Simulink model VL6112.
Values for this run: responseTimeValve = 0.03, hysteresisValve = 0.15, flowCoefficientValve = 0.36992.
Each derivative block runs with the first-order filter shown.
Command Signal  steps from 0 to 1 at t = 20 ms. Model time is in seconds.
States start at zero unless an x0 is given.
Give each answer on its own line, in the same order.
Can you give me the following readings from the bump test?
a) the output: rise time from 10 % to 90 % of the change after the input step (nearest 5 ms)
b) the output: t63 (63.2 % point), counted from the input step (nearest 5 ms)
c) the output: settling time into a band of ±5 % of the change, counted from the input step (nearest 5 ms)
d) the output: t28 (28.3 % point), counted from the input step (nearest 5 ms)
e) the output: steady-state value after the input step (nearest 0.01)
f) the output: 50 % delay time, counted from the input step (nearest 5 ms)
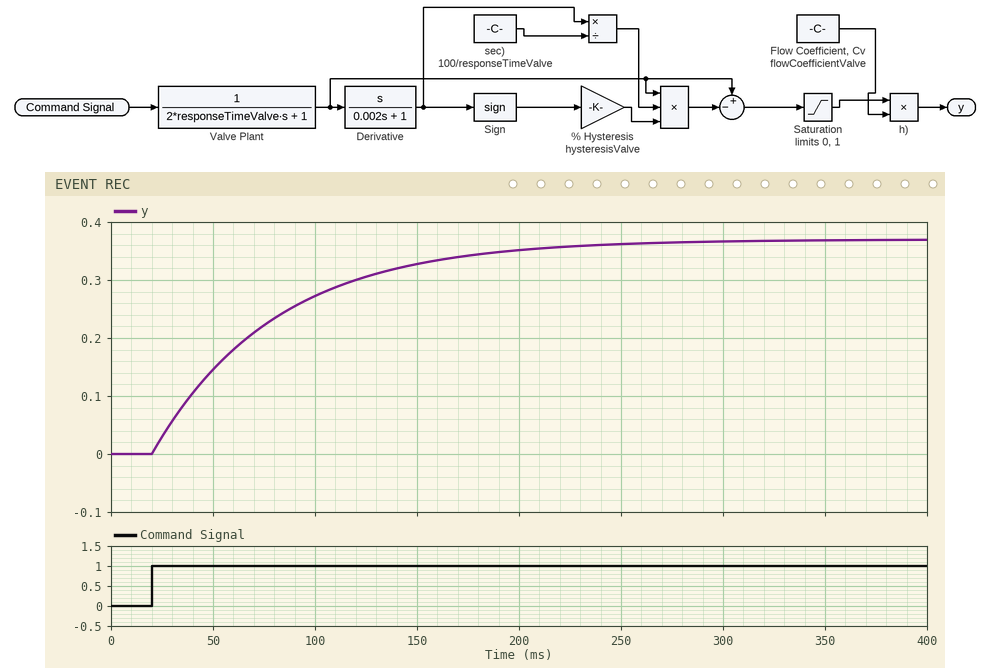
130 ms
60 ms
180 ms
20 ms
0.37
40 ms
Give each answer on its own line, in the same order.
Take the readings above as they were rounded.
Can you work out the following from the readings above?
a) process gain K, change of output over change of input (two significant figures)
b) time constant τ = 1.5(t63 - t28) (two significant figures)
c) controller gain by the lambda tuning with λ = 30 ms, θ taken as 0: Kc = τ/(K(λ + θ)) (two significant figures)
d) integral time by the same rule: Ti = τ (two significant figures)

0.37
60 ms
5.4
60 ms
